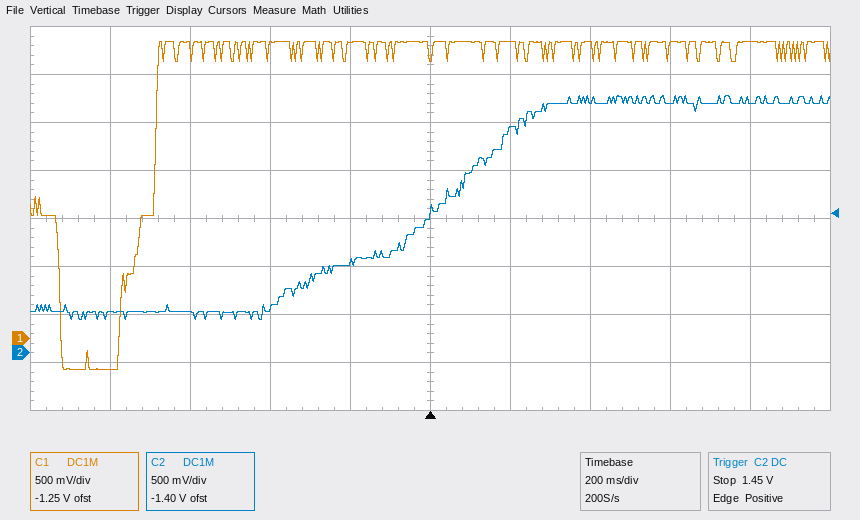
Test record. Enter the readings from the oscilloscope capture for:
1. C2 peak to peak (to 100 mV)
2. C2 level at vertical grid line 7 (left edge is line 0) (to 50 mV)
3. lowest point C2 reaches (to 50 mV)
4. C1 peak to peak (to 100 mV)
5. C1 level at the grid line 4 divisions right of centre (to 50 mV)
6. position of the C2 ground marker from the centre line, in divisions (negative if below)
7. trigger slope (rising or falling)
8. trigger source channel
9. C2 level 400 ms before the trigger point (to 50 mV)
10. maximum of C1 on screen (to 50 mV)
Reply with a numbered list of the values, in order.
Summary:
1. 2.30 V
2. 2.65 V
3. 350 mV
4. 3.40 V
5. 3.10 V
6. -2.8 div
7. rising
8. C2
9. 450 mV
10. 3.10 V
